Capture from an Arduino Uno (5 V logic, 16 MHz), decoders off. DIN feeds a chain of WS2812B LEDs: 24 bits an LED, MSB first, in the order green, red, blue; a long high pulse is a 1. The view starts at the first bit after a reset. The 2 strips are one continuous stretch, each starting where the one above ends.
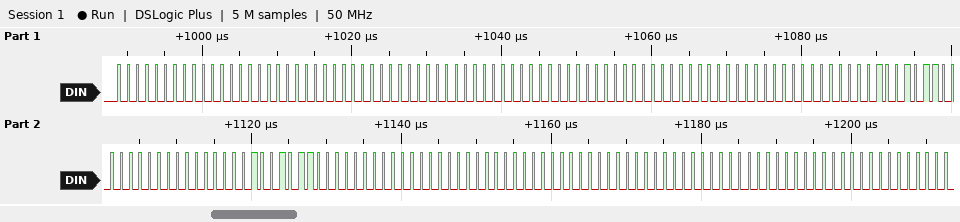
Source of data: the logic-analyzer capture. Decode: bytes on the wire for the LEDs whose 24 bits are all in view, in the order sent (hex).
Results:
00 00 00 00 00 00 00 00 00 00 4B 00 00 4B 00 00 00 00 00 00 00
